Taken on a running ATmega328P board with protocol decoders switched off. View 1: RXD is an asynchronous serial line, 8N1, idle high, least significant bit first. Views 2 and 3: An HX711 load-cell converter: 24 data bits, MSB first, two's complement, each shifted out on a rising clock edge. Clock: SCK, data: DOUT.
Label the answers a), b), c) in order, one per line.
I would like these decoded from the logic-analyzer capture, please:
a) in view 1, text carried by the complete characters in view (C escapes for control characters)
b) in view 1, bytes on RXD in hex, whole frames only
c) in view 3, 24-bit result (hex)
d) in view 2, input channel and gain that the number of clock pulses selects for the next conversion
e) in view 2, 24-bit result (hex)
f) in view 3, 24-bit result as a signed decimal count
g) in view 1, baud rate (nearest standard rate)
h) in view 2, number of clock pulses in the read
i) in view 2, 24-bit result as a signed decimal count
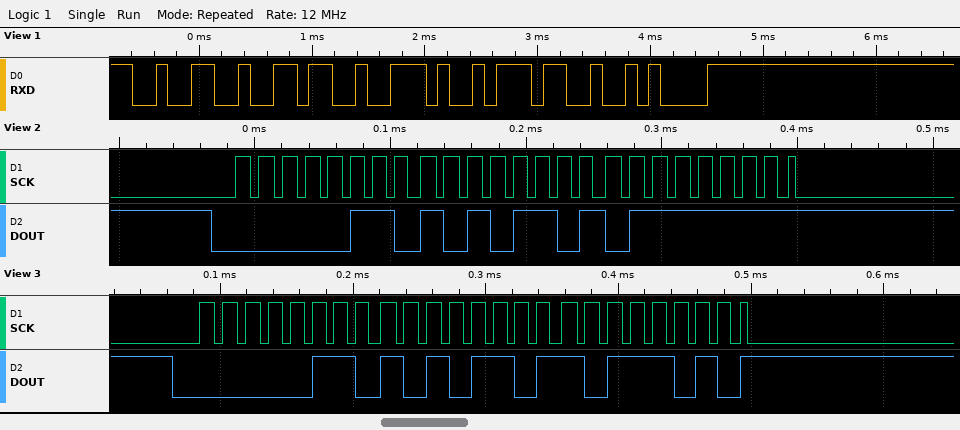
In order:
a) "26.7\n"
b) 32 36 2E 37 0A
c) 0x06ADBA
d) channel A, gain 128
e) 0x06AD7F
f) 437690
g) 9600 baud
h) 25
i) 437631
